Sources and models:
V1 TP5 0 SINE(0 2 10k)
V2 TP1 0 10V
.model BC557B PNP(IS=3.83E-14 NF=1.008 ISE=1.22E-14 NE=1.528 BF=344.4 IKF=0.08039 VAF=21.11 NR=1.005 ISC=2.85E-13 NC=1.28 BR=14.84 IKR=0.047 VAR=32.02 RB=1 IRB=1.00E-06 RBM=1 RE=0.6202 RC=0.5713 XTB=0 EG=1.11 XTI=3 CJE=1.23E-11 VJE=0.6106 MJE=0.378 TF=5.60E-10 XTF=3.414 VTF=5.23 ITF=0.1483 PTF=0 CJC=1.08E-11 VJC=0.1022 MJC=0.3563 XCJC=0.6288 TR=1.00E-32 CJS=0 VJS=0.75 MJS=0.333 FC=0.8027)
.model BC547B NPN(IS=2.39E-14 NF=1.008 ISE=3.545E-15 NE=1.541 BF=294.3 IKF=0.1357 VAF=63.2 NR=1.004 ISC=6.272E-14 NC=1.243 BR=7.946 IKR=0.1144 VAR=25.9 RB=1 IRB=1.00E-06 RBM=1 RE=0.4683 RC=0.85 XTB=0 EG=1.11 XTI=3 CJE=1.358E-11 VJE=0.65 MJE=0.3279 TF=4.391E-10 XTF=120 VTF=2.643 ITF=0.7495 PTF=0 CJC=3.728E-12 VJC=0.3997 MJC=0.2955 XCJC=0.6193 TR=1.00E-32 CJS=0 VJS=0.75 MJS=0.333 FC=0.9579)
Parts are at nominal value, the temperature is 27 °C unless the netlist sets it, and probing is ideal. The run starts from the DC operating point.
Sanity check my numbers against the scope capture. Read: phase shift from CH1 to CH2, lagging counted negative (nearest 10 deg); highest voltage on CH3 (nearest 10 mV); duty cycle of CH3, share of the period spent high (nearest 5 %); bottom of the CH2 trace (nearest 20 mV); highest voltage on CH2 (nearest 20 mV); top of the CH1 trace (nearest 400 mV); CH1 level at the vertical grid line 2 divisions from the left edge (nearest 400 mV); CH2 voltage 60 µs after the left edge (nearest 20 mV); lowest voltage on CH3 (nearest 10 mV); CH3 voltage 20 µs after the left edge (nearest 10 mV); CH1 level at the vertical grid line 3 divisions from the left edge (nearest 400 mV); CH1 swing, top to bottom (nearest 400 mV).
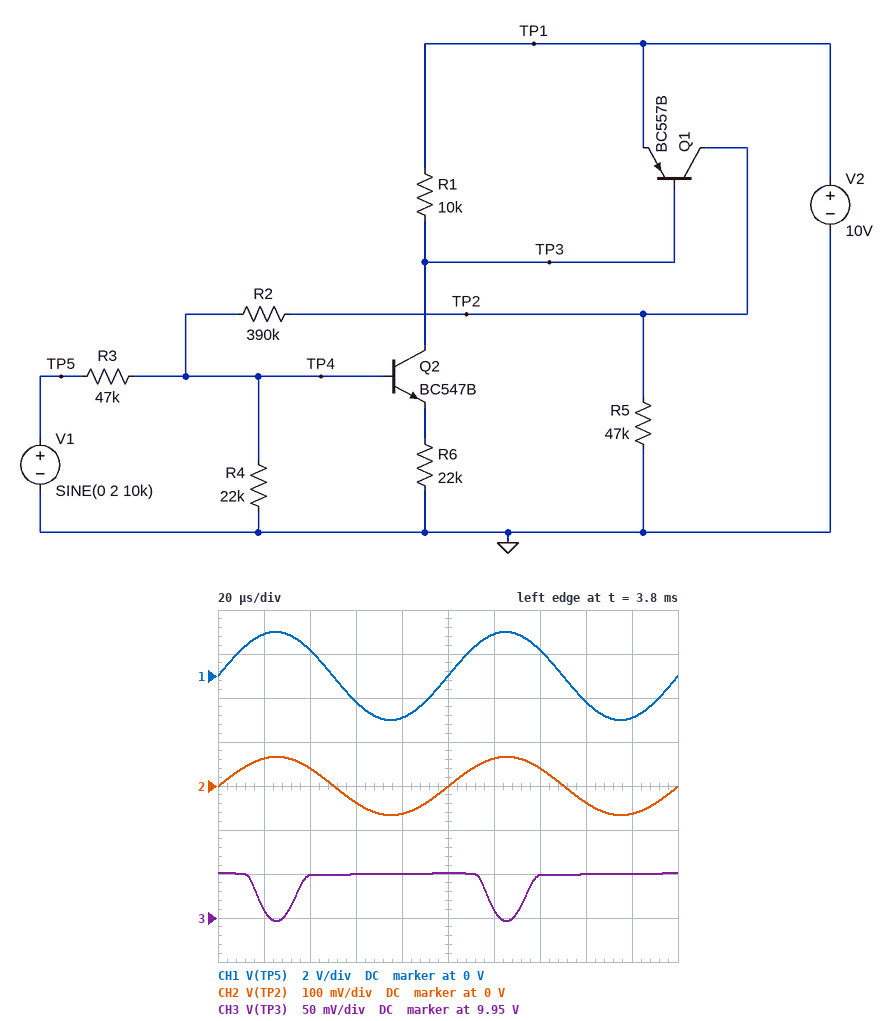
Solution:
0 deg
10.00 V
85 %
-60 mV
60 mV
2.0 V
1.2 V
-40 mV
9.95 V
9.96 V
-1.2 V
4.0 V
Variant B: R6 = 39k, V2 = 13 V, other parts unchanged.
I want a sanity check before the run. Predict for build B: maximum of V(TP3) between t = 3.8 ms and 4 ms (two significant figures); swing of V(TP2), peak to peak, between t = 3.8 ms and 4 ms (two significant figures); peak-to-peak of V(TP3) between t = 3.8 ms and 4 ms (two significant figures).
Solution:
13 V
130 mV
34 mV
